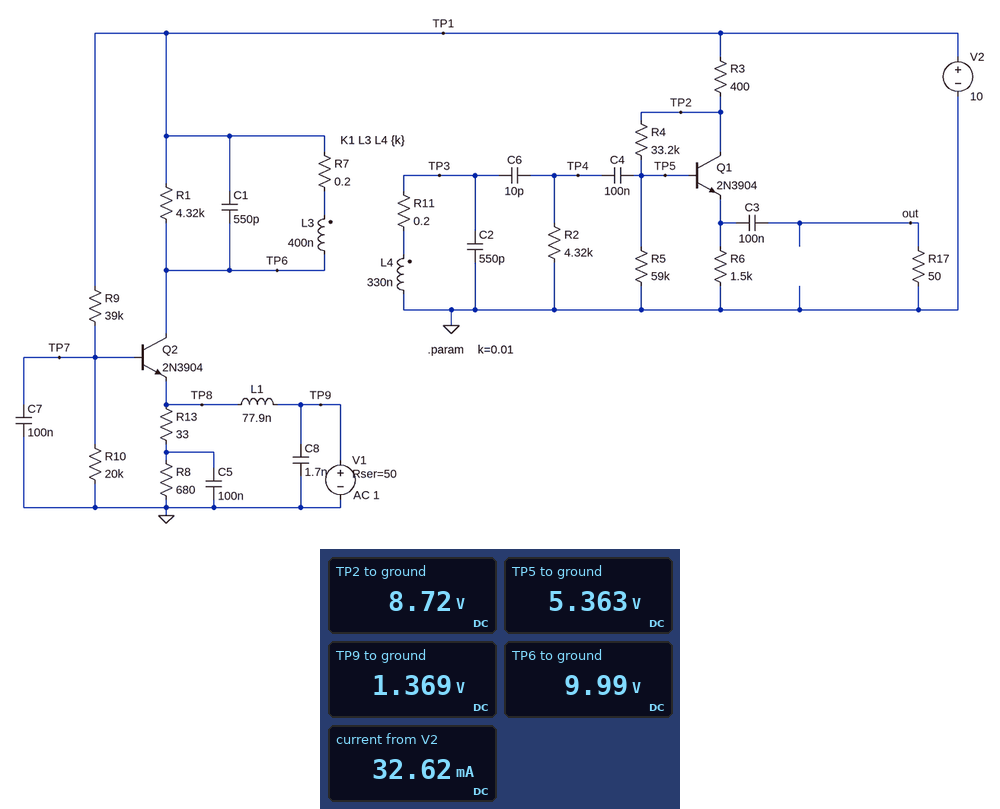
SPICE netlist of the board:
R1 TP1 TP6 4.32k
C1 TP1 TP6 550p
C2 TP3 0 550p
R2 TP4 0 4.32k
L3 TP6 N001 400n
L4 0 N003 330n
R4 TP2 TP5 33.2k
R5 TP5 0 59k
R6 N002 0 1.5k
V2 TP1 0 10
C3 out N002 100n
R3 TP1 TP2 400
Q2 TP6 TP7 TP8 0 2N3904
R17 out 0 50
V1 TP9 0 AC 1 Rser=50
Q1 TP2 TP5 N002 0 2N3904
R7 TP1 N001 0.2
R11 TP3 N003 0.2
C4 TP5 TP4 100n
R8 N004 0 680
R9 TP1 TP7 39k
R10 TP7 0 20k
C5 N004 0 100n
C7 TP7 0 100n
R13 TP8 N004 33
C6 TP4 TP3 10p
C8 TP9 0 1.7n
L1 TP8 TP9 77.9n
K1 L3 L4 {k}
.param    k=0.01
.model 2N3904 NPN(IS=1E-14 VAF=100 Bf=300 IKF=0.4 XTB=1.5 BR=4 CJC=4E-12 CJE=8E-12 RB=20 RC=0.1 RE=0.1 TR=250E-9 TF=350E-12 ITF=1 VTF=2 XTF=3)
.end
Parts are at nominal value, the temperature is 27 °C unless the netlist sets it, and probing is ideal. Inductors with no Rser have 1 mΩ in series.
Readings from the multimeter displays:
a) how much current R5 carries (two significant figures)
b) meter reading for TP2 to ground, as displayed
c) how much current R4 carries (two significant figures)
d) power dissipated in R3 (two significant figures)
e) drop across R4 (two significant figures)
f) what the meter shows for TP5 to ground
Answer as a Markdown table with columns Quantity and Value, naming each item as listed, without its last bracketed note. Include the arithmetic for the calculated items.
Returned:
| Quantity | Value |
|---|---|
| how much current R5 carries | (5.363 V) / 59 kΩ = 91 µA |
| meter reading for TP2 to ground, as displayed | 8.72 V |
| how much current R4 carries | (8.72 V - 5.363 V) / 33.2 kΩ = 100 µA |
| power dissipated in R3 | (10 V - 8.72 V)^2 / 400 Ω = 4.1 mW |
| drop across R4 | 8.72 V - 5.363 V = 3.4 V |
| what the meter shows for TP5 to ground | 5.363 V |
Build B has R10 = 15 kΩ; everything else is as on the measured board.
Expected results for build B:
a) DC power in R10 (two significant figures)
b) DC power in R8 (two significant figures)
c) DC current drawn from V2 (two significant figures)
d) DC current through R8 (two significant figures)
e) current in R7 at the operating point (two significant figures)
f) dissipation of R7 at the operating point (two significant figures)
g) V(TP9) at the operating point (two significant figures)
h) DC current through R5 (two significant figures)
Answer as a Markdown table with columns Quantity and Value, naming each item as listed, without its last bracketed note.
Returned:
| Quantity | Value |
|---|---|
| DC power in R10 | 240 µW |
| DC power in R8 | 1.8 mW |
| DC current drawn from V2 | 28 mA |
| DC current through R8 | 1.6 mA |
| current in R7 at the operating point | 25 mA |
| dissipation of R7 at the operating point | 120 µW |
| V(TP9) at the operating point | 1.2 V |
| DC current through R5 | 91 µA |
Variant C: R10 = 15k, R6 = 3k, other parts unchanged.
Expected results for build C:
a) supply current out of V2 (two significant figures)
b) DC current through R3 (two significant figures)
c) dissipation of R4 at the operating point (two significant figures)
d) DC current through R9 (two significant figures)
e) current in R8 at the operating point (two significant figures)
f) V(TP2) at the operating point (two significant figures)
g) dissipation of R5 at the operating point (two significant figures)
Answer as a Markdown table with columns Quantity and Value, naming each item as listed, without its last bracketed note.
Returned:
| Quantity | Value |
|---|---|
| supply current out of V2 | 27 mA |
| DC current through R3 | 1.8 mA |
| dissipation of R4 at the operating point | 360 µW |
| DC current through R9 | 210 µA |
| current in R8 at the operating point | 1.6 mA |
| V(TP2) at the operating point | 9.3 V |
| dissipation of R5 at the operating point | 570 µW |
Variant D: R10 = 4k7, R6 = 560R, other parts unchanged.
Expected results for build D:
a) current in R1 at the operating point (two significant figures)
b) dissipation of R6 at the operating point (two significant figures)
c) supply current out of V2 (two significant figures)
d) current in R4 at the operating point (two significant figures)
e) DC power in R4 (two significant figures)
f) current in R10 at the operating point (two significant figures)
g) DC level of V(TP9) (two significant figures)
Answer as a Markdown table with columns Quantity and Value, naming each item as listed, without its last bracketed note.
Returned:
| Quantity | Value |
|---|---|
| current in R1 at the operating point | 290 nA |
| dissipation of R6 at the operating point | 23 mW |
| supply current out of V2 | 13 mA |
| current in R4 at the operating point | 94 µA |
| DC power in R4 | 290 µW |
| current in R10 at the operating point | 210 µA |
| DC level of V(TP9) | 290 mV |
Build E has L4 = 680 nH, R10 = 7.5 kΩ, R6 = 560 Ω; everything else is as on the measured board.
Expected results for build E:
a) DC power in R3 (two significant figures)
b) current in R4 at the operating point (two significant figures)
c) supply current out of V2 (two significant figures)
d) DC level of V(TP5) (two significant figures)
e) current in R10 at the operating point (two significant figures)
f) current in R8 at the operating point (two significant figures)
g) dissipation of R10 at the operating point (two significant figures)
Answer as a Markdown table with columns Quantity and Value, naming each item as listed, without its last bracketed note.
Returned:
| Quantity | Value |
|---|---|
| DC power in R3 | 17 mW |
| current in R4 at the operating point | 94 µA |
| supply current out of V2 | 20 mA |
| DC level of V(TP5) | 4.3 V |
| current in R10 at the operating point | 180 µA |
| current in R8 at the operating point | 880 µA |
| dissipation of R10 at the operating point | 240 µW |
